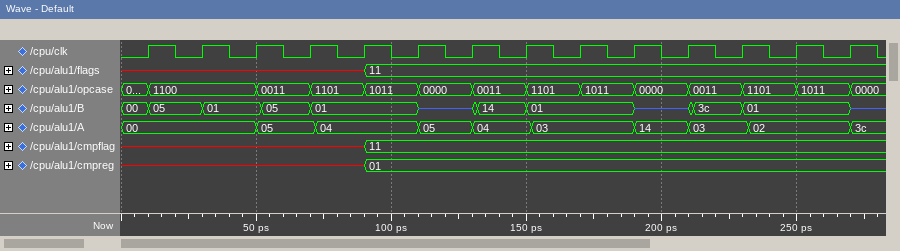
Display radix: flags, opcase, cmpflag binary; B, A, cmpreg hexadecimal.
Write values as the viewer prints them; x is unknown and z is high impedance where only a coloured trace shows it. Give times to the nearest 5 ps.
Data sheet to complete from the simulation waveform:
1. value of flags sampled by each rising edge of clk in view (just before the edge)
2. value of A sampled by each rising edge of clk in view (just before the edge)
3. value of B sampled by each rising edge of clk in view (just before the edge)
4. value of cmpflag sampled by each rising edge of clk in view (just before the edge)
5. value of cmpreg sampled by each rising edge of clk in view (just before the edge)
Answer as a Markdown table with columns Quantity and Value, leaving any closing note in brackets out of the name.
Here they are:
| Quantity | Value |
|---|---|
| value of flags sampled by each rising edge of clk in view | x, x, x, x, x, 11, 11, 11, 11, 11, 11, 11, 11, 11 |
| value of A sampled by each rising edge of clk in view | 00, 00, 00, 05, 04, 04, 05, 04, 03, 03, 14, 03, 02, 02 |
| value of B sampled by each rising edge of clk in view | 00, 05, 01, 05, 01, 01, z, 14, 01, 01, z, 3c, 01, 01 |
| value of cmpflag sampled by each rising edge of clk in view | x, x, x, x, x, 11, 11, 11, 11, 11, 11, 11, 11, 11 |
| value of cmpreg sampled by each rising edge of clk in view | x, x, x, x, x, 01, 01, 01, 01, 01, 01, 01, 01, 01 |
